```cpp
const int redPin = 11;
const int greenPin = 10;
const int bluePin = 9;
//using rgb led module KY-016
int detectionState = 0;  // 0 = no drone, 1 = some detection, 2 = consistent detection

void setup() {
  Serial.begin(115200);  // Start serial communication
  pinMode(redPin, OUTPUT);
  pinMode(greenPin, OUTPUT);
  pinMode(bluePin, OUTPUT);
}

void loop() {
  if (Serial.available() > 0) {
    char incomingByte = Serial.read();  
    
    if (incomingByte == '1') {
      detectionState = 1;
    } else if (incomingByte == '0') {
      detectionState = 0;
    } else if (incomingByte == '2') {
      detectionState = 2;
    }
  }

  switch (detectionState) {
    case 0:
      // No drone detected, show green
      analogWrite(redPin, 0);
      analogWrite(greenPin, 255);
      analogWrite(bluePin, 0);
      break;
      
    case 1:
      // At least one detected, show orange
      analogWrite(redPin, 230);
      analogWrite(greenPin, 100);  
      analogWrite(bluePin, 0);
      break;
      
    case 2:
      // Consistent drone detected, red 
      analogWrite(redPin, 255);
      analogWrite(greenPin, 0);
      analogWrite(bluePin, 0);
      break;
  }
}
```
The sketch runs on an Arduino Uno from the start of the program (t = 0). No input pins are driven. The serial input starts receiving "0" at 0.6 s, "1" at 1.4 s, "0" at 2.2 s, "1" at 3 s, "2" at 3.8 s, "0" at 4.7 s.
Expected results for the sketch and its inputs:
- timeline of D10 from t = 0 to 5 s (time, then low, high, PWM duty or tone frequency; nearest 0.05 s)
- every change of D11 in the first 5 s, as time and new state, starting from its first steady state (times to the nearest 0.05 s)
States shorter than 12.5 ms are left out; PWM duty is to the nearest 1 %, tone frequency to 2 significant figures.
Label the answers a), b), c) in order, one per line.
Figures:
a) 0 s high; 1.4 s PWM 39 %; 2.2 s high; 3 s PWM 39 %; 3.8 s low; 4.7 s high
b) 0 s low; 1.4 s PWM 90 %; 2.2 s low; 3 s PWM 90 %; 3.8 s high; 4.7 s low
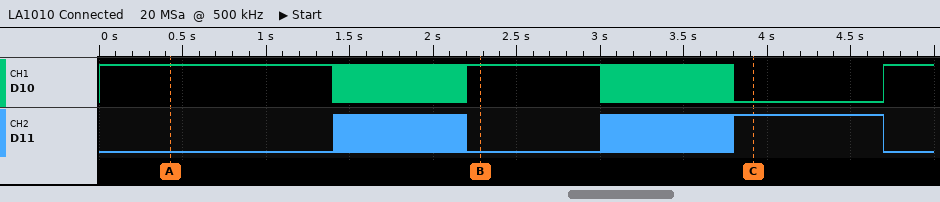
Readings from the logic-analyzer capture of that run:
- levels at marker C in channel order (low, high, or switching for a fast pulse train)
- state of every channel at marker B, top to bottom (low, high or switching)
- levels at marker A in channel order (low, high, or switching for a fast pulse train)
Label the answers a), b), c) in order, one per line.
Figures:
a) D10 low, D11 high
b) D10 high, D11 low
c) D10 high, D11 low
